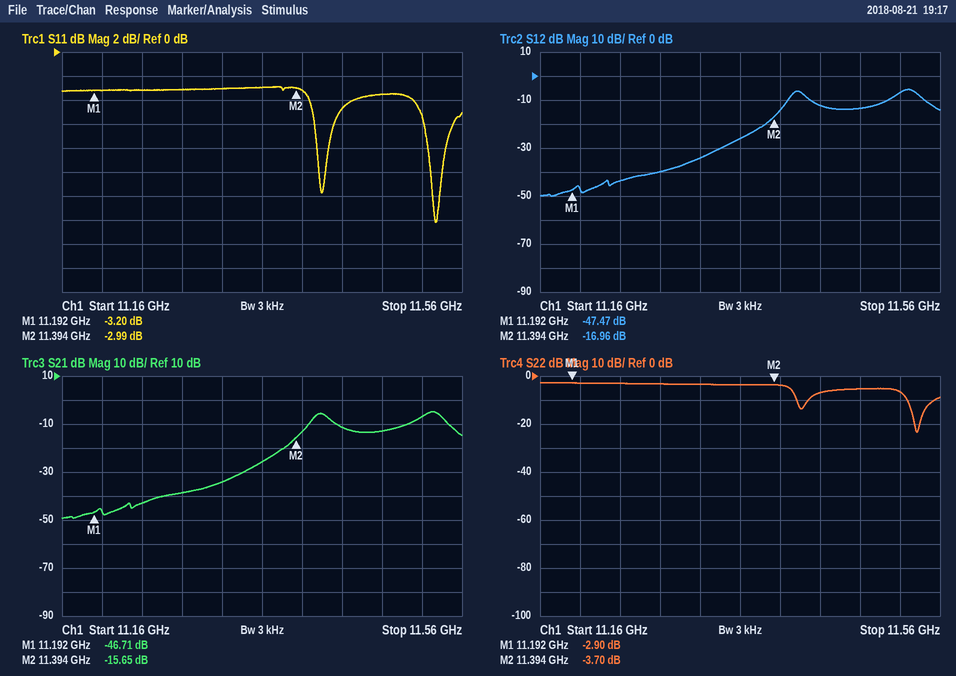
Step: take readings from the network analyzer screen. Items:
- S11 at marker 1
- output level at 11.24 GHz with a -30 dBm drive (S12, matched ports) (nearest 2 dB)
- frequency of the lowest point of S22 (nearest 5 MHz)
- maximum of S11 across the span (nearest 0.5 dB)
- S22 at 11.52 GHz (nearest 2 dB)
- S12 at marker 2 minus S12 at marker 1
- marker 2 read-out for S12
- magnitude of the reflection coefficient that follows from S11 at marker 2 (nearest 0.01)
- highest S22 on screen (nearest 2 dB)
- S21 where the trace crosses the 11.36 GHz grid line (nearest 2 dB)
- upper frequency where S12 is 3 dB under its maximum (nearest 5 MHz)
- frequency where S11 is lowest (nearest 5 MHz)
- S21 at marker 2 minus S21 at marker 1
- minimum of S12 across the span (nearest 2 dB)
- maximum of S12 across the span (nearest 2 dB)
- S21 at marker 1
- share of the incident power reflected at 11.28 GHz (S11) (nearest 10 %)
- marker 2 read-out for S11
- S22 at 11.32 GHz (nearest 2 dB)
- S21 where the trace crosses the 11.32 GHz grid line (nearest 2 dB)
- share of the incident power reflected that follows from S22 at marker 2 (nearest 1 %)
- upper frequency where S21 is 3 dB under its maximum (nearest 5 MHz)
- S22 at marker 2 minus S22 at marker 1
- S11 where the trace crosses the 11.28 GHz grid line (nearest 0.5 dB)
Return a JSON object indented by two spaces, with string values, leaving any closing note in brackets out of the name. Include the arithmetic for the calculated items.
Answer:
{
  "S11 at marker 1": "-3.20 dB",
  "output level at 11.24 GHz with a -30 dBm drive (S12, matched ports)": "-30 dBm + (-44 dB) = -74 dBm",
  "frequency of the lowest point of S22": "11.535 GHz",
  "maximum of S11 across the span": "-3.0 dB",
  "S22 at 11.52 GHz": "-6 dB",
  "S12 at marker 2 minus S12 at marker 1": "-16.96 − (-47.47) = 30.51 dB",
  "marker 2 read-out for S12": "-16.96 dB",
  "magnitude of the reflection coefficient that follows from S11 at marker 2": "10^(-2.99/20) ≈ 0.71",
  "highest S22 on screen": "-2 dB",
  "S21 where the trace crosses the 11.36 GHz grid line": "-26 dB",
  "upper frequency where S12 is 3 dB under its maximum": "11.540 GHz",
  "frequency where S11 is lowest": "11.535 GHz",
  "S21 at marker 2 minus S21 at marker 1": "-15.65 − (-46.71) = 31.06 dB",
  "minimum of S12 across the span": "-50 dB",
  "maximum of S12 across the span": "-6 dB",
  "S21 at marker 1": "-46.71 dB",
  "share of the incident power reflected at 11.28 GHz (S11)": "10^(-3/10) ≈ 50 %",
  "marker 2 read-out for S11": "-2.99 dB",
  "S22 at 11.32 GHz": "-4 dB",
  "S21 where the trace crosses the 11.32 GHz grid line": "-34 dB",
  "share of the incident power reflected that follows from S22 at marker 2": "10^(-3.7/10) ≈ 43 %",
  "upper frequency where S21 is 3 dB under its maximum": "11.540 GHz",
  "S22 at marker 2 minus S22 at marker 1": "-3.7 − (-2.9) = -0.80 dB",
  "S11 where the trace crosses the 11.28 GHz grid line": "-3.0 dB"
}
